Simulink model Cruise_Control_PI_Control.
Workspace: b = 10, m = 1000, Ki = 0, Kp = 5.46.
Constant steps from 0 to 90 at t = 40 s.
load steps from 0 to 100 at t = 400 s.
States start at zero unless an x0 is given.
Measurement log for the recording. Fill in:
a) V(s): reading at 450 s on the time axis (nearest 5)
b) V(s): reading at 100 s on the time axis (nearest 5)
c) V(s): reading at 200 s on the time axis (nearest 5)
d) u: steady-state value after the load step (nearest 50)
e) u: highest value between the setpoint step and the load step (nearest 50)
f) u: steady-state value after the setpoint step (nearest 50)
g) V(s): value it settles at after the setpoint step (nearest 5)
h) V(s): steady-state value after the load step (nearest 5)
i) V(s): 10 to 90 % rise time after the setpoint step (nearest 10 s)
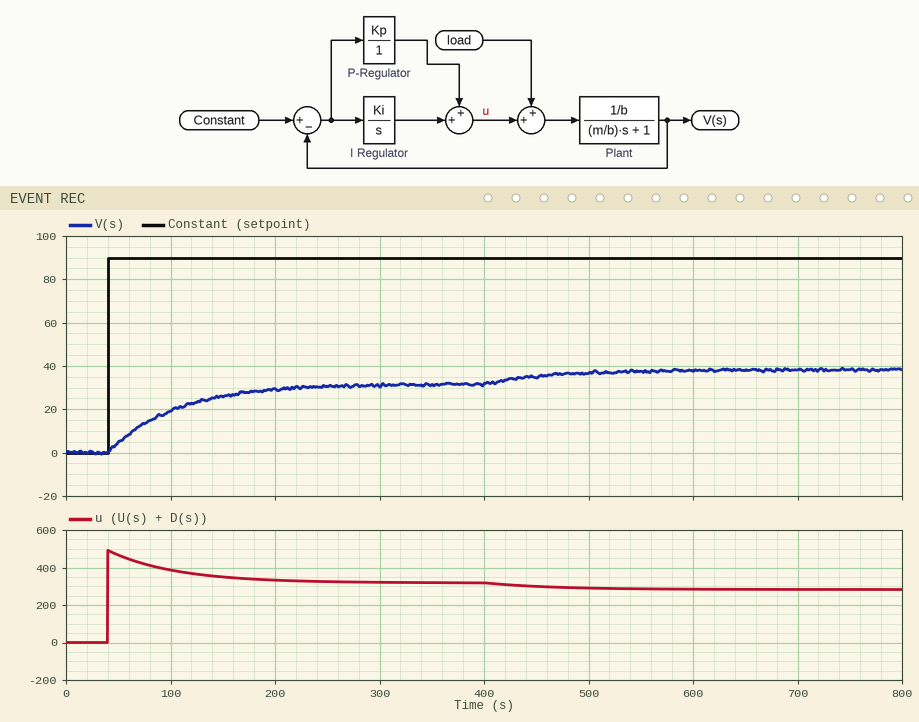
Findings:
35
20
30
300
500
300
30
40
140 s
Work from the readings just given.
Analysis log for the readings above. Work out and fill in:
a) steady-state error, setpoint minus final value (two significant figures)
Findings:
60
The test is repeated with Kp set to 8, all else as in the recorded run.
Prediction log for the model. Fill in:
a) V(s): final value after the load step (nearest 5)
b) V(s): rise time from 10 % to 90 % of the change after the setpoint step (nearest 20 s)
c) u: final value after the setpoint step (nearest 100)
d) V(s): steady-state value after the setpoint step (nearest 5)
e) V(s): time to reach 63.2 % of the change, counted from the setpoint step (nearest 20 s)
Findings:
45
120 s
400
40
60 s
